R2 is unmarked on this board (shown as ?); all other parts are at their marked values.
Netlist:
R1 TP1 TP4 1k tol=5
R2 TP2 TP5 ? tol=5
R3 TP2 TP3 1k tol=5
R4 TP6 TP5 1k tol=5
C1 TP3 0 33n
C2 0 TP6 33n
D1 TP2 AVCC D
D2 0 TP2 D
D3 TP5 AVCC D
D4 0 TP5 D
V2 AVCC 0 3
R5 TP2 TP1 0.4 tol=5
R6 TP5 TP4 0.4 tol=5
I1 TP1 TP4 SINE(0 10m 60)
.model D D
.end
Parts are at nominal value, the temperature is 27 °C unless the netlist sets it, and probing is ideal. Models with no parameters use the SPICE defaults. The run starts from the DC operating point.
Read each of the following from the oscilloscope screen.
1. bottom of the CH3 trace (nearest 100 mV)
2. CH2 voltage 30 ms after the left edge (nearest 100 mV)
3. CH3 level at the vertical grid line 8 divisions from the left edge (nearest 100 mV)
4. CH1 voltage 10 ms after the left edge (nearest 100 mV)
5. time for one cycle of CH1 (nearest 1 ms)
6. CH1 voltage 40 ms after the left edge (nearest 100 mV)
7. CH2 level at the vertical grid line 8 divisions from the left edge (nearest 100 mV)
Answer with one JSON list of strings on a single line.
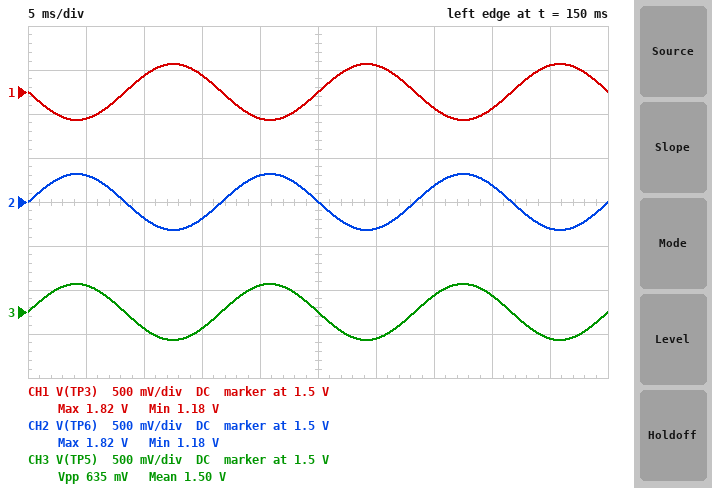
["1.2 V", "1.2 V", "1.7 V", "1.7 V", "17 ms", "1.3 V", "1.7 V"]
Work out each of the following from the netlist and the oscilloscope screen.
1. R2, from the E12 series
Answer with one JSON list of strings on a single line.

["68 Ω"]
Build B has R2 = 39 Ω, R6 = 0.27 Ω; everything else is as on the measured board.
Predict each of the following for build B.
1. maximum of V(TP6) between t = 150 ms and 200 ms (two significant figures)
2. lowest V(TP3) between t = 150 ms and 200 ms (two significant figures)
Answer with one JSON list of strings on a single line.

["1.7 V", "1.3 V"]
